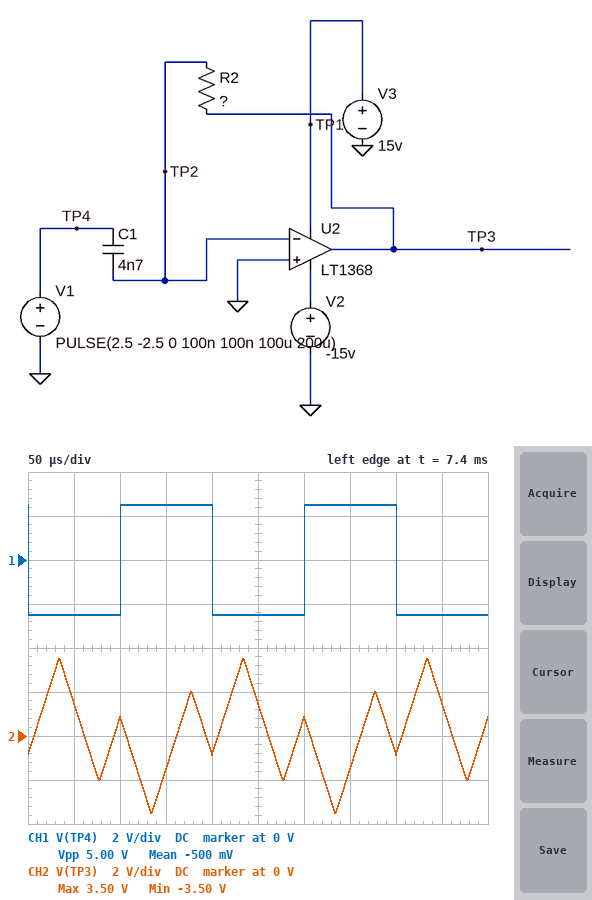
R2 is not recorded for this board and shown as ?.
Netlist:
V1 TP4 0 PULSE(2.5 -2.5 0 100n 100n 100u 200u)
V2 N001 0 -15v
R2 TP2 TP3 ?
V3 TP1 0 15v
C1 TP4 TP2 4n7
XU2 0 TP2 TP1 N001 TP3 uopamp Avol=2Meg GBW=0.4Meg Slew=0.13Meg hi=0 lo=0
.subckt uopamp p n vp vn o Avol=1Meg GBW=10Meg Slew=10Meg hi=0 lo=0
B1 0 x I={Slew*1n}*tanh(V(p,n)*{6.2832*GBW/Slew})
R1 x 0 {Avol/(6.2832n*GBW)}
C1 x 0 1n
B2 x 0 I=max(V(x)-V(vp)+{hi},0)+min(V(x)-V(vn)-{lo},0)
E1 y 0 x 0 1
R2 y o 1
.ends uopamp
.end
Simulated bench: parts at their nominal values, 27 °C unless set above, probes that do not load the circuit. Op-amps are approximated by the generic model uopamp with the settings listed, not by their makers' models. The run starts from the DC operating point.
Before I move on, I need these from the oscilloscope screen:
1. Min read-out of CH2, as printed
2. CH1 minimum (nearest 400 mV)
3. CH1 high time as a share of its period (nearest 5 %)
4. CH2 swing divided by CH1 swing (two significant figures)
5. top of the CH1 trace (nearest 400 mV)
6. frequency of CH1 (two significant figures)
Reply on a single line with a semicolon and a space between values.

-3.50 V; -2.4 V; 50 %; 1.4; 2.4 V; 5.0 kHz
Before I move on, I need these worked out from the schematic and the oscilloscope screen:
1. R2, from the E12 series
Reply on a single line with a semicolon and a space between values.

5.6 kΩ
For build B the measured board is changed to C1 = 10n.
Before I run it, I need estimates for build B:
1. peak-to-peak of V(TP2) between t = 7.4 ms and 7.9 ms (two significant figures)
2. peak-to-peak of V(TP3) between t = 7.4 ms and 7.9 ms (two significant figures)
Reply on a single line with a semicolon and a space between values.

14 V; 13 V
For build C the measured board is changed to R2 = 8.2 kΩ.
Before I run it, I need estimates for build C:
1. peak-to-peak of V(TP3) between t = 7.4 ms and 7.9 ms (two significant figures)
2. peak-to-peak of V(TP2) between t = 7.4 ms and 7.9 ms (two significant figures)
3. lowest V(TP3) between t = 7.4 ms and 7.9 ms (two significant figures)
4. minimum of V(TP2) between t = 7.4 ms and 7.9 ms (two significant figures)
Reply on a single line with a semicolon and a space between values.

13 V; 11 V; -6.5 V; -5.5 V
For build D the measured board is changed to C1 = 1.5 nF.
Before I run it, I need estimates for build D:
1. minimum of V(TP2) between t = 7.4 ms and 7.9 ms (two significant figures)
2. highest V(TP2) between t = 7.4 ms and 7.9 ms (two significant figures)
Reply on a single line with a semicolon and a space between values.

-5.0 V; 5.0 V
